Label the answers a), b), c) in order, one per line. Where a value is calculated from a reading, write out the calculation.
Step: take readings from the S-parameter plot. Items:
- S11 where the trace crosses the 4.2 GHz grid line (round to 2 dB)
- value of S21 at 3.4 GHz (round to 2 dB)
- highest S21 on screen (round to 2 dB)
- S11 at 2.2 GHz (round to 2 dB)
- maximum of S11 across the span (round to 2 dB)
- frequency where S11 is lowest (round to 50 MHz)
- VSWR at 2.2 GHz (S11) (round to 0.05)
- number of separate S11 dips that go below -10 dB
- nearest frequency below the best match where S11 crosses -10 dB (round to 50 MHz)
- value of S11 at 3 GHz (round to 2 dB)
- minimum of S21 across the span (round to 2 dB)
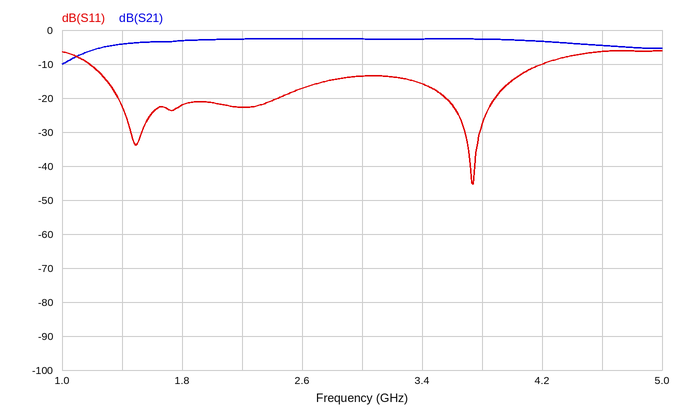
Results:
a) -10 dB
b) -2 dB
c) -2 dB
d) -22 dB
e) -6 dB
f) 3.75 GHz
g) |Γ| = 10^(-22/20) = 0.0794; VSWR = (1 + 0.0794)/(1 − 0.0794) ≈ 1.17, so 1.15 to the nearest 0.05
h) 2
i) 1.20 GHz
j) -14 dB
k) -10 dB
